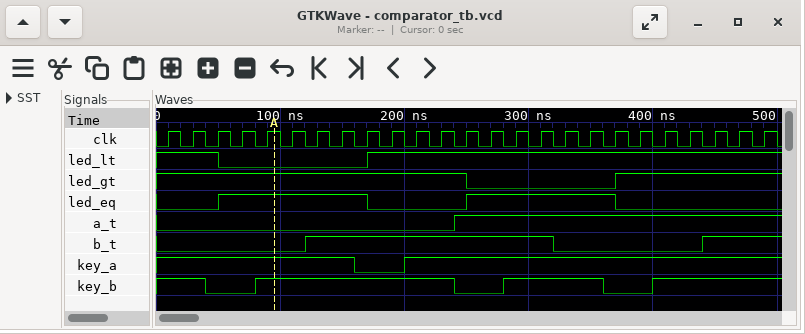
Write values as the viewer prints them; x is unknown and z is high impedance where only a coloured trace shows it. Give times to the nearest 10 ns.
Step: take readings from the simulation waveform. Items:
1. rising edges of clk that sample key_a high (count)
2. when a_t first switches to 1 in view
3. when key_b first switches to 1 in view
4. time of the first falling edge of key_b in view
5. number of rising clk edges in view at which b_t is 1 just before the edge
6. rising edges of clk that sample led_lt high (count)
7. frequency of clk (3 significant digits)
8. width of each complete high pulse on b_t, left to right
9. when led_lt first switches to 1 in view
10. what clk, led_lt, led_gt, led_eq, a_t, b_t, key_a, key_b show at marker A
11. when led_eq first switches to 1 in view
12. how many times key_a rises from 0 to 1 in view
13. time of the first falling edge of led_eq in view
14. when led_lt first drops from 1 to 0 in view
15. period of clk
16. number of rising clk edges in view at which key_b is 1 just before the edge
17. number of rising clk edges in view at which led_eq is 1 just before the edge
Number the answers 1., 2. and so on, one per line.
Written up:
1. 23
2. 240 ns
3. 80 ns
4. 40 ns
5. 13
6. 19
7. 50.0 MHz
8. 200 ns
9. 170 ns
10. clk=1, led_lt=0, led_gt=1, led_eq=1, a_t=0, b_t=0, key_a=1, key_b=1
11. 50 ns
12. 1
13. 170 ns
14. 50 ns
15. 20 ns
16. 19
17. 12
